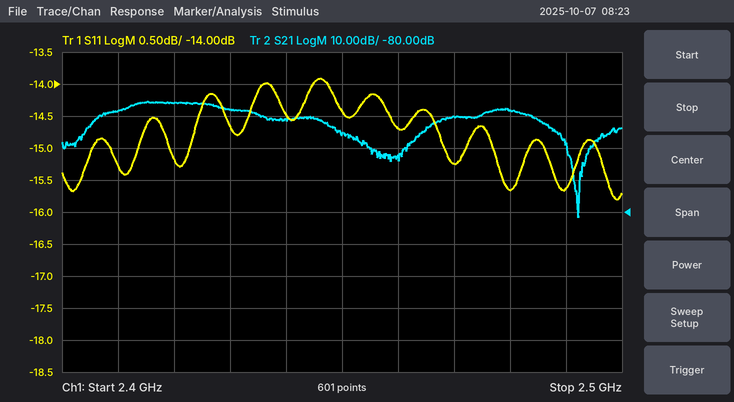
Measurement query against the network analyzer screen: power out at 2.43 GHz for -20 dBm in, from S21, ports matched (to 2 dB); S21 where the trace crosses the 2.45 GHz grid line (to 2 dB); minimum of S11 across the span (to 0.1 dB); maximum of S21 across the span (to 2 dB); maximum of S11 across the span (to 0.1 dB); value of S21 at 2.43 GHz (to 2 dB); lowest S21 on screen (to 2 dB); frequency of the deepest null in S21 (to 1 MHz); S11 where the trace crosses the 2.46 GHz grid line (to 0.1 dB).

-68 dBm
-56 dB
-15.8 dB
-46 dB
-13.9 dB
-48 dB
-82 dB
2.492 GHz
-14.7 dB
